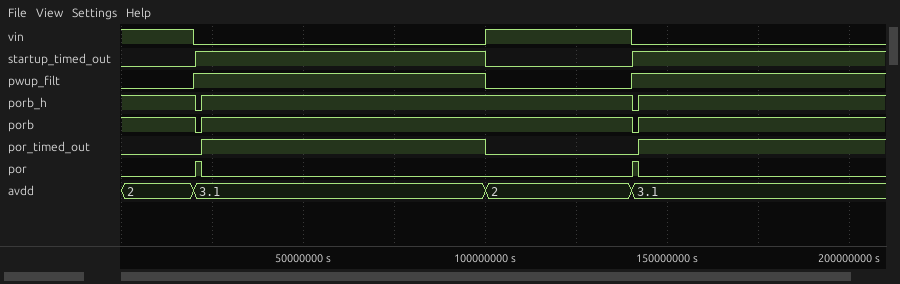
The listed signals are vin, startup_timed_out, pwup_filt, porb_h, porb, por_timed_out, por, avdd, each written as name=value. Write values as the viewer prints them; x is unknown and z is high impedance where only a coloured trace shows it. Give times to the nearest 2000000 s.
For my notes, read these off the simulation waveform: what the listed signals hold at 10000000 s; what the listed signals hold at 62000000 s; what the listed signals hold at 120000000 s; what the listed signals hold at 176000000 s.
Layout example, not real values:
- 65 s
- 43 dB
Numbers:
- vin=1, startup_timed_out=0, pwup_filt=0, porb_h=1, porb=1, por_timed_out=0, por=0, avdd=2
- vin=0, startup_timed_out=1, pwup_filt=1, porb_h=1, porb=1, por_timed_out=1, por=0, avdd=3.1
- vin=1, startup_timed_out=0, pwup_filt=0, porb_h=1, porb=1, por_timed_out=0, por=0, avdd=2
- vin=0, startup_timed_out=1, pwup_filt=1, porb_h=1, porb=1, por_timed_out=1, por=0, avdd=3.1
